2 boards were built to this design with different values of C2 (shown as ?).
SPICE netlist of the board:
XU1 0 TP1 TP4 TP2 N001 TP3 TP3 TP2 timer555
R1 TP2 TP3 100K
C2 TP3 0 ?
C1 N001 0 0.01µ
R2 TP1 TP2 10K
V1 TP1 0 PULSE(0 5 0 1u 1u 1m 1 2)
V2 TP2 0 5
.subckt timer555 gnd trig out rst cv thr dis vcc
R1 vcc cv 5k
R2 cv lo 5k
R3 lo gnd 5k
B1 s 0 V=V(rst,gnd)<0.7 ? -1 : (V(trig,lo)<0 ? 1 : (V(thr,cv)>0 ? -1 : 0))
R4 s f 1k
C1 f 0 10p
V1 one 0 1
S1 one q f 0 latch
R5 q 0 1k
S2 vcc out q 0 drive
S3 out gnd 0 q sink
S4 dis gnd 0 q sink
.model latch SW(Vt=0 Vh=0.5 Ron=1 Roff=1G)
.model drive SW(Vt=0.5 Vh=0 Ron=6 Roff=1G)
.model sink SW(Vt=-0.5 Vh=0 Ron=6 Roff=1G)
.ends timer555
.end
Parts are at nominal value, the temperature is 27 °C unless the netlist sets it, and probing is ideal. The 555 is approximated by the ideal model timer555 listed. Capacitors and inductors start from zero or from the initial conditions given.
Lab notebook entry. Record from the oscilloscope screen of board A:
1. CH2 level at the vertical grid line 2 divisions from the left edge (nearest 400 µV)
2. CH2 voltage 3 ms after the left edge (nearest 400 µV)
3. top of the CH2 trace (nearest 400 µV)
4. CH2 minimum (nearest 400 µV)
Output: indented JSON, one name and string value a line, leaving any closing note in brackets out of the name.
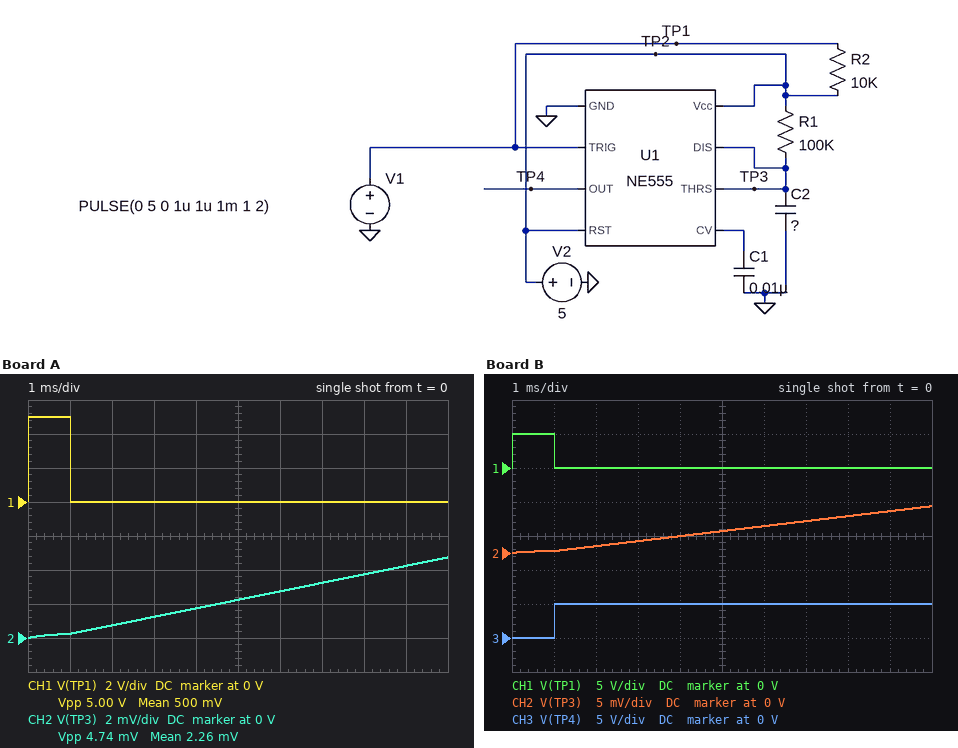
{
  "CH2 level at the vertical grid line 2 divisions from the left edge": "800 µV",
  "CH2 voltage 3 ms after the left edge": "1.2 mV",
  "top of the CH2 trace": "4.8 mV",
  "CH2 minimum": "0 V"
}
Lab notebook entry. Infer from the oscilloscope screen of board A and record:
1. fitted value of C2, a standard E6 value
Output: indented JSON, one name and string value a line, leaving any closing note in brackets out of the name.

{
  "fitted value of C2, a standard E6 value": "100 µF"
}
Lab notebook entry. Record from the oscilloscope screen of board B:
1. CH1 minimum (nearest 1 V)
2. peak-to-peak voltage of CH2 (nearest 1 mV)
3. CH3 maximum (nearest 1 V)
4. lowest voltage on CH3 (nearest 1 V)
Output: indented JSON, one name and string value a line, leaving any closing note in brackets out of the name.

{
  "CH1 minimum": "0 V",
  "peak-to-peak voltage of CH2": "7 mV",
  "CH3 maximum": "5 V",
  "lowest voltage on CH3": "0 V"
}
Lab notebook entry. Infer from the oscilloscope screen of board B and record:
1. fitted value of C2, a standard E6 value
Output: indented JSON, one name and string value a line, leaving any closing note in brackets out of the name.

{
  "fitted value of C2, a standard E6 value": "68 µF"
}
